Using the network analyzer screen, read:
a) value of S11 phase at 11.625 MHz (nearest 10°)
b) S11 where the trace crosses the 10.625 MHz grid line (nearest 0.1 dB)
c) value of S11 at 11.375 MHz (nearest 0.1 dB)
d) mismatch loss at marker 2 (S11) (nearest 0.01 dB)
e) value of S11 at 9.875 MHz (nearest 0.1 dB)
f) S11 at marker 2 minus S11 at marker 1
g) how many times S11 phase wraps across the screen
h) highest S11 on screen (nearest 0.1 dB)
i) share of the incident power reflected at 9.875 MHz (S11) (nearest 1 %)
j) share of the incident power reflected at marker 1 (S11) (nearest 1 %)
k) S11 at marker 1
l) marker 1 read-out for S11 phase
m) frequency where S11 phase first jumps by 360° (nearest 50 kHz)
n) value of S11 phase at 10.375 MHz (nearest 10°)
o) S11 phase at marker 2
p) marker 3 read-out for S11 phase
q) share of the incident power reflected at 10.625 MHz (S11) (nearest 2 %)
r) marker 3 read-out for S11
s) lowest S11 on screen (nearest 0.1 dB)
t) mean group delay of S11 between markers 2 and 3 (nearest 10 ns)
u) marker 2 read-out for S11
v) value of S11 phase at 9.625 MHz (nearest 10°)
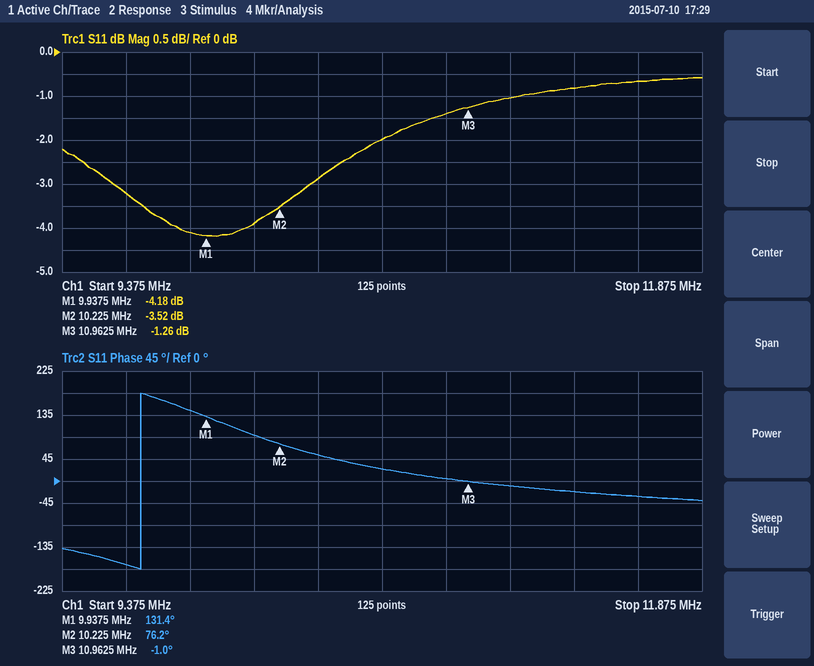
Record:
-30°
-2.0 dB
-0.8 dB
2.55 dB
-4.1 dB
0.66 dB
1
-0.6 dB
39 %
38 %
-4.18 dB
131.4°
9.70 MHz
50°
76.2°
-1.0°
64 %
-1.26 dB
-4.2 dB
290 ns
-3.52 dB
-170°
